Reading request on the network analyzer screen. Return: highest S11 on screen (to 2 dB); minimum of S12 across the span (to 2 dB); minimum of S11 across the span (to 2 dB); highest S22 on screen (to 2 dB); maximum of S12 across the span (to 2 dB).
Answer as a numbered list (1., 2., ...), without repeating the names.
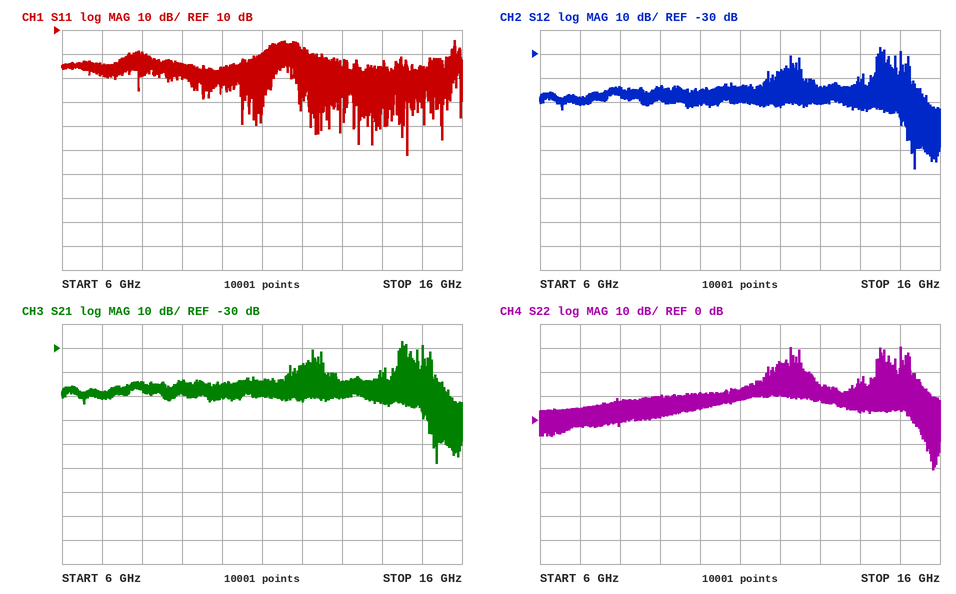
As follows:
1. 6 dB
2. -78 dB
3. -42 dB
4. 30 dB
5. -28 dB
